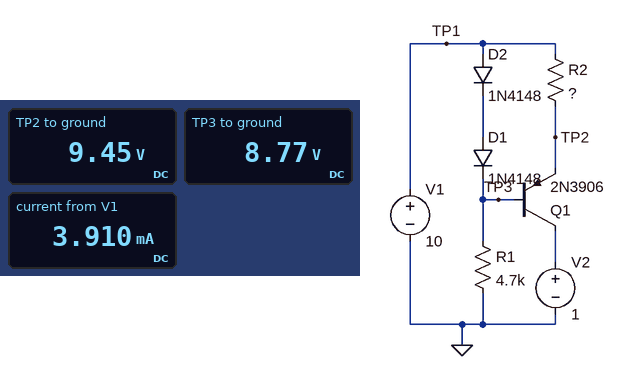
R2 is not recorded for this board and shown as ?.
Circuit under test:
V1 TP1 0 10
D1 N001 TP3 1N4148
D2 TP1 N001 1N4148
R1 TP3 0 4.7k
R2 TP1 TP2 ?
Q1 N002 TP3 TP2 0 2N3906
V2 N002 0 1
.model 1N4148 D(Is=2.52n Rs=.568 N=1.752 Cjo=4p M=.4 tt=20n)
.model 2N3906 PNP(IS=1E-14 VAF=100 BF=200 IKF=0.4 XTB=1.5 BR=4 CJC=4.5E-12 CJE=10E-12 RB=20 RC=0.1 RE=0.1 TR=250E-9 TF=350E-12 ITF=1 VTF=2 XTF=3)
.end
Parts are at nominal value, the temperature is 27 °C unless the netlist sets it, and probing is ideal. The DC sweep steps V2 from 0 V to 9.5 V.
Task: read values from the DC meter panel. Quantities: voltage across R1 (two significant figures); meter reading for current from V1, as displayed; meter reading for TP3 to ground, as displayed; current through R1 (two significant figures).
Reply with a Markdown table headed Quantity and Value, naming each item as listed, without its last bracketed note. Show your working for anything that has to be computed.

| Quantity | Value |
|---|---|
| voltage across R1 | 8.77 V = 8.8 V |
| meter reading for current from V1, as displayed | 3.910 mA |
| meter reading for TP3 to ground, as displayed | 8.77 V |
| current through R1 | (8.77 V) / 4.7 kΩ = 1.9 mA |
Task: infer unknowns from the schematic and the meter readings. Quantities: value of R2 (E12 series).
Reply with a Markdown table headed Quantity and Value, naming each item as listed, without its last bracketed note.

| Quantity | Value |
|---|---|
| value of R2 | 270 Ω |
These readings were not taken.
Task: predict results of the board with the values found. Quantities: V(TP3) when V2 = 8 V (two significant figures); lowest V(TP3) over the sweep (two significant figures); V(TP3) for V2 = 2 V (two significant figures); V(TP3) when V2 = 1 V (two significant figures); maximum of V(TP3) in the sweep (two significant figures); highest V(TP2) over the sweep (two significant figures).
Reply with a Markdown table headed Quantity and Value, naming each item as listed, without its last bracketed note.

| Quantity | Value |
|---|---|
| V(TP3) when V2 = 8 V | 8.8 V |
| lowest V(TP3) over the sweep | 8.8 V |
| V(TP3) for V2 = 2 V | 8.8 V |
| V(TP3) when V2 = 1 V | 8.8 V |
| maximum of V(TP3) in the sweep | 8.8 V |
| highest V(TP2) over the sweep | 9.5 V |
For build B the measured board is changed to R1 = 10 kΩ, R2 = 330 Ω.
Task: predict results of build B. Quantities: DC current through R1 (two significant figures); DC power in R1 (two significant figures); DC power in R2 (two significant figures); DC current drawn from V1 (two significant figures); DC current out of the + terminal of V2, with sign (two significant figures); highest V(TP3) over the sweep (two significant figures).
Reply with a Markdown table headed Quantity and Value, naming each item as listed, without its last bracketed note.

| Quantity | Value |
|---|---|
| DC current through R1 | 880 µA |
| DC power in R1 | 7.8 mW |
| DC power in R2 | 740 µW |
| DC current drawn from V1 | 2.4 mA |
| DC current out of the + terminal of V2, with sign | -1.5 mA |
| highest V(TP3) over the sweep | 8.9 V |
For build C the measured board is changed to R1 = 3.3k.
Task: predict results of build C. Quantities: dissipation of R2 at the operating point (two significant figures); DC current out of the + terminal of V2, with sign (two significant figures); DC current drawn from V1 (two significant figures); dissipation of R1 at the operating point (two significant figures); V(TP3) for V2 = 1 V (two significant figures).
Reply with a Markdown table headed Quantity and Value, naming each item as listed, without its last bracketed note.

| Quantity | Value |
|---|---|
| dissipation of R2 at the operating point | 1.3 mW |
| DC current out of the + terminal of V2, with sign | -2.2 mA |
| DC current drawn from V1 | 4.8 mA |
| dissipation of R1 at the operating point | 23 mW |
| V(TP3) for V2 = 1 V | 8.7 V |
